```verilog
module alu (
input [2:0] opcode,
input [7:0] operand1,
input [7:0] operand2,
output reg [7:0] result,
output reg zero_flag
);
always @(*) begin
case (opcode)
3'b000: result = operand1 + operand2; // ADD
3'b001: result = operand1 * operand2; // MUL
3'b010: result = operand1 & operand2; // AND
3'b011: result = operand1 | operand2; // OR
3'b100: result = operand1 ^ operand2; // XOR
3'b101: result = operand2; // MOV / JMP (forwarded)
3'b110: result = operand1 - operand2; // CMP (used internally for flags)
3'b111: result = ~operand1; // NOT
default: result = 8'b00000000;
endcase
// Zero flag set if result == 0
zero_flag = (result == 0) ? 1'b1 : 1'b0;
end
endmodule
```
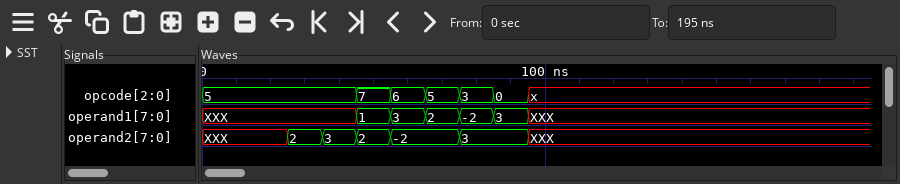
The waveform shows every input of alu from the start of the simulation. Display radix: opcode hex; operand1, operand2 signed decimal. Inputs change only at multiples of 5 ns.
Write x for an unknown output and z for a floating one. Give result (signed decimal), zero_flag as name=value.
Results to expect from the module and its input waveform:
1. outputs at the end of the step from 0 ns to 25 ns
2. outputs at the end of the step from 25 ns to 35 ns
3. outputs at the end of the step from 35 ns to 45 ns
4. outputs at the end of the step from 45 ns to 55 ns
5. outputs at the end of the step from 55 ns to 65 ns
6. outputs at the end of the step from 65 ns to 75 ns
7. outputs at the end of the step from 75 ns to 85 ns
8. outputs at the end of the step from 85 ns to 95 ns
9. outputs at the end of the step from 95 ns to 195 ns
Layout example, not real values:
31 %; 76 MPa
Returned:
result=x, zero_flag=x; result=2, zero_flag=0; result=3, zero_flag=0; result=-2, zero_flag=0; result=5, zero_flag=0; result=-2, zero_flag=0; result=-1, zero_flag=0; result=6, zero_flag=0; result=0, zero_flag=1
